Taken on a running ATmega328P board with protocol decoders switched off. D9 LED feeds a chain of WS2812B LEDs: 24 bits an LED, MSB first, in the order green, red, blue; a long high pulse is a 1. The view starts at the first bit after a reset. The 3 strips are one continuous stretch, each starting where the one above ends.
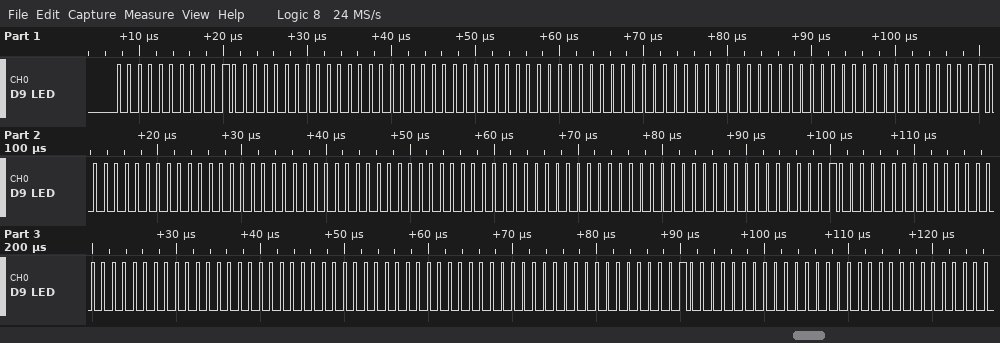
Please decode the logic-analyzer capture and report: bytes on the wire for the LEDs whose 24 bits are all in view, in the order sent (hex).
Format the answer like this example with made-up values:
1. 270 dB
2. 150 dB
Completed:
1. 00 20 00 00 00 00 00 00 00 00 20 00 00 00 00 00 00 00 00 20 00 00 00 00 00 00 00 00 20 00
